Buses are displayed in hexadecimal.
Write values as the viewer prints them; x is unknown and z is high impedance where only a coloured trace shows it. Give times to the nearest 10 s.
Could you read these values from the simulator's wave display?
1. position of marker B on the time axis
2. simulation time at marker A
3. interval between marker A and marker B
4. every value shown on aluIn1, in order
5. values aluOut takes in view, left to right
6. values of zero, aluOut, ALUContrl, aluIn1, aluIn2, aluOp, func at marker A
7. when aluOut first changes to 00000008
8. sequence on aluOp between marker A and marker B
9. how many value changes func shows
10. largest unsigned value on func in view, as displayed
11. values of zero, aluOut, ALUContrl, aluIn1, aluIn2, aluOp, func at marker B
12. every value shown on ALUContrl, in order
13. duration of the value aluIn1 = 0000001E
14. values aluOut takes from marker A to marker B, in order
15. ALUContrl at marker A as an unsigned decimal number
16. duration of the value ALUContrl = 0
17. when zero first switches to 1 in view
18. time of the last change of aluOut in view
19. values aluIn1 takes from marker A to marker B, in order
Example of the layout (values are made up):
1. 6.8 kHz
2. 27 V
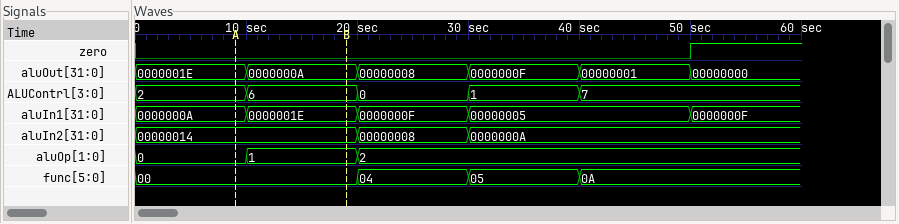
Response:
1. 20 s
2. 10 s
3. 10 s
4. 0000000A, 0000001E, 0000000F, 00000005, 0000000F
5. 0000001E, 0000000A, 00000008, 0000000F, 00000001, 00000000
6. zero=0, aluOut=0000001E, ALUContrl=2, aluIn1=0000000A, aluIn2=00000014, aluOp=0, func=00
7. 20 s
8. 0, 1
9. 3
10. 0A
11. zero=0, aluOut=0000000A, ALUContrl=6, aluIn1=0000001E, aluIn2=00000014, aluOp=1, func=00
12. 2, 6, 0, 1, 7
13. 10 s
14. 0000001E, 0000000A
15. 2
16. 10 s
17. 50 s
18. 50 s
19. 0000000A, 0000001E
